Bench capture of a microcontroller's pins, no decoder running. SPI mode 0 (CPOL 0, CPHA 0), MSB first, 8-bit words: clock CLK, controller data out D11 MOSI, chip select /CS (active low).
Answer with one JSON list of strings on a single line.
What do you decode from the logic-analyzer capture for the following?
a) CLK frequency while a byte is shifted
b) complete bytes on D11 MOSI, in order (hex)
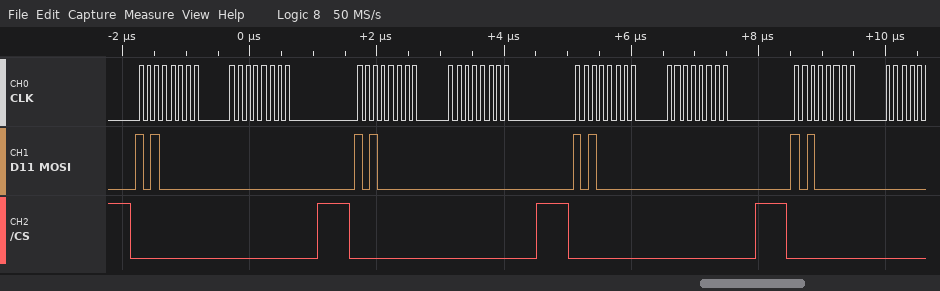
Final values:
["8 MHz", "A0 00 A0 00 A0 00 A0"]
